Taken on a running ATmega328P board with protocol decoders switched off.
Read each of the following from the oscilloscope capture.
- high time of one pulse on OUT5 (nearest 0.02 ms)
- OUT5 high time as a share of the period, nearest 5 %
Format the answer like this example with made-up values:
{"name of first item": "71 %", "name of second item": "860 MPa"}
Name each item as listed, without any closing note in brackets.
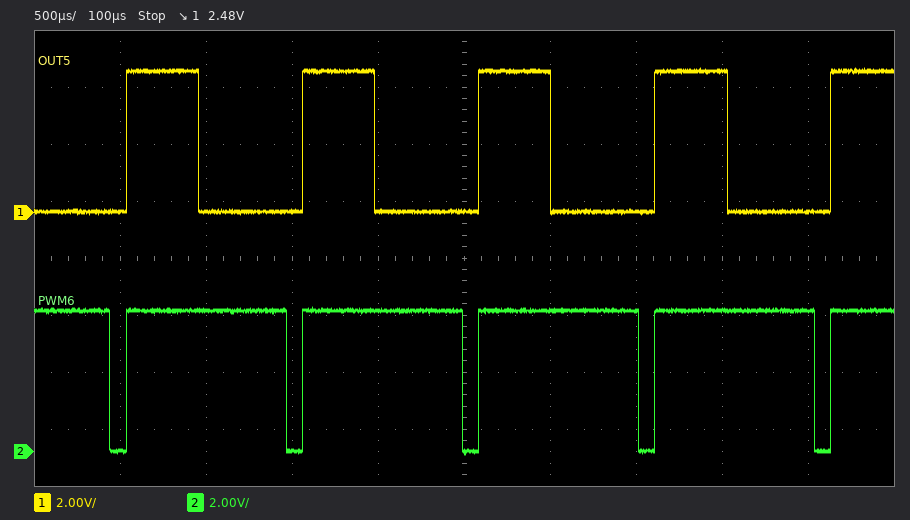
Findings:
{"high time of one pulse on OUT5": "0.42 ms", "OUT5 high time as a share of the period, nearest 5 %": "40 %"}
